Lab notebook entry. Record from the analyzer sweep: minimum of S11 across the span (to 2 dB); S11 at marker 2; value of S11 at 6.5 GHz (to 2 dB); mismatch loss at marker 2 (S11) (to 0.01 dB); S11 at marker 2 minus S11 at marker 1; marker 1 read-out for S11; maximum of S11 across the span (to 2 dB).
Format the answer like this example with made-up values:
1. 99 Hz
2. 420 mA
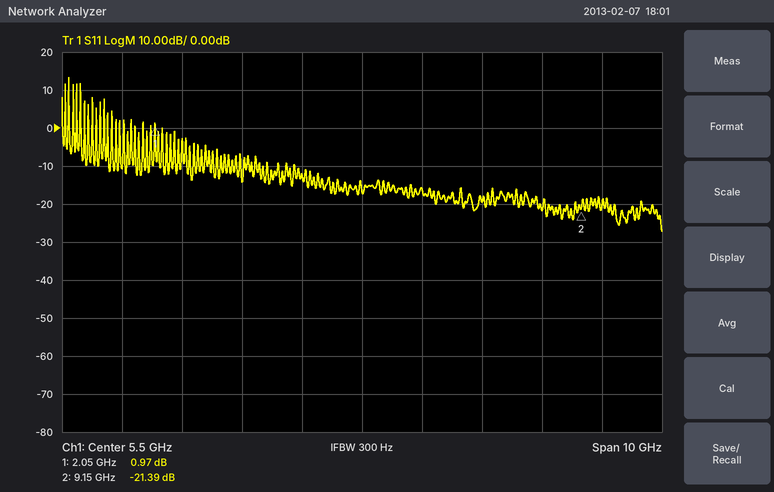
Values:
1. -28 dB
2. -21.39 dB
3. -16 dB
4. 0.03 dB
5. -22.36 dB
6. 0.97 dB
7. 14 dB
